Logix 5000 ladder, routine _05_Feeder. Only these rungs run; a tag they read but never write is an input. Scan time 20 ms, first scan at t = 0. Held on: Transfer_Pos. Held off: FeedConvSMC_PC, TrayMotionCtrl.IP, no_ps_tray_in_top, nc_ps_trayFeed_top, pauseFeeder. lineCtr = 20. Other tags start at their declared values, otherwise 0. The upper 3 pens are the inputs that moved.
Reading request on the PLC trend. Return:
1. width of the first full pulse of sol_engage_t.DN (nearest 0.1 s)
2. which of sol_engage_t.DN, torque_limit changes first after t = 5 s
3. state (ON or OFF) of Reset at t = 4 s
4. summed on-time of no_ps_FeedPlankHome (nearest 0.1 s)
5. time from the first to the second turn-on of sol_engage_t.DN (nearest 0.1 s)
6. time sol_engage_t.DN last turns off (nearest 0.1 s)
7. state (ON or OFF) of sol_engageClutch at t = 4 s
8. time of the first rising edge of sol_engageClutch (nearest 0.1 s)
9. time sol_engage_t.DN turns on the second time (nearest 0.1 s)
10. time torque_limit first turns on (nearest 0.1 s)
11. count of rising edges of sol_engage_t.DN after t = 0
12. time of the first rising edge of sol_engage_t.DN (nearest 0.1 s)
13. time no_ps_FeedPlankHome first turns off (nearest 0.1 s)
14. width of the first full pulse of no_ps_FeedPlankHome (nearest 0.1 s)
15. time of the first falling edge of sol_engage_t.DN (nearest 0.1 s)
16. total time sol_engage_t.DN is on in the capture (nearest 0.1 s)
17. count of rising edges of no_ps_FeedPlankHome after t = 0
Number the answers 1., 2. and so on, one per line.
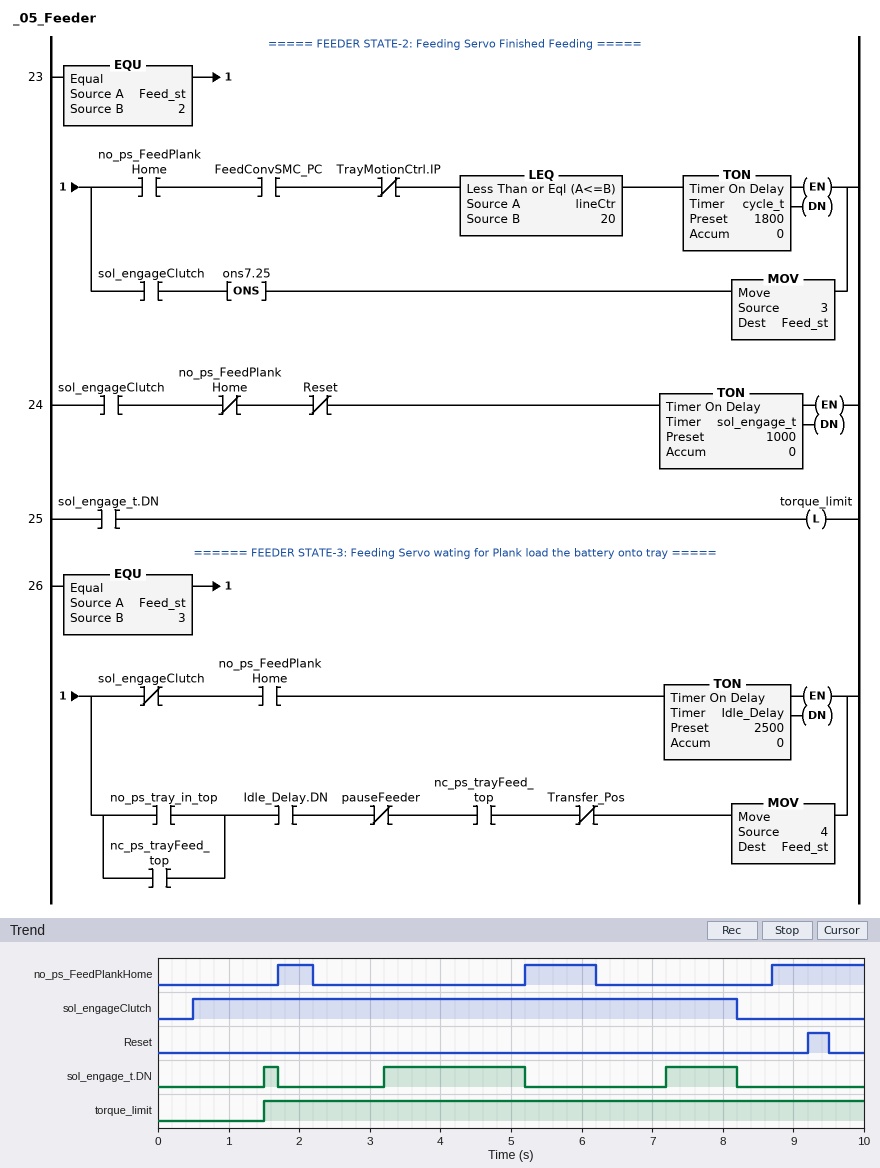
1. 0.2 s
2. sol_engage_t.DN
3. OFF
4. 2.8 s
5. 1.7 s
6. 8.2 s
7. ON
8. 0.5 s
9. 3.2 s
10. 1.5 s
11. 3
12. 1.5 s
13. 2.2 s
14. 0.5 s
15. 1.7 s
16. 3.2 s
17. 3
